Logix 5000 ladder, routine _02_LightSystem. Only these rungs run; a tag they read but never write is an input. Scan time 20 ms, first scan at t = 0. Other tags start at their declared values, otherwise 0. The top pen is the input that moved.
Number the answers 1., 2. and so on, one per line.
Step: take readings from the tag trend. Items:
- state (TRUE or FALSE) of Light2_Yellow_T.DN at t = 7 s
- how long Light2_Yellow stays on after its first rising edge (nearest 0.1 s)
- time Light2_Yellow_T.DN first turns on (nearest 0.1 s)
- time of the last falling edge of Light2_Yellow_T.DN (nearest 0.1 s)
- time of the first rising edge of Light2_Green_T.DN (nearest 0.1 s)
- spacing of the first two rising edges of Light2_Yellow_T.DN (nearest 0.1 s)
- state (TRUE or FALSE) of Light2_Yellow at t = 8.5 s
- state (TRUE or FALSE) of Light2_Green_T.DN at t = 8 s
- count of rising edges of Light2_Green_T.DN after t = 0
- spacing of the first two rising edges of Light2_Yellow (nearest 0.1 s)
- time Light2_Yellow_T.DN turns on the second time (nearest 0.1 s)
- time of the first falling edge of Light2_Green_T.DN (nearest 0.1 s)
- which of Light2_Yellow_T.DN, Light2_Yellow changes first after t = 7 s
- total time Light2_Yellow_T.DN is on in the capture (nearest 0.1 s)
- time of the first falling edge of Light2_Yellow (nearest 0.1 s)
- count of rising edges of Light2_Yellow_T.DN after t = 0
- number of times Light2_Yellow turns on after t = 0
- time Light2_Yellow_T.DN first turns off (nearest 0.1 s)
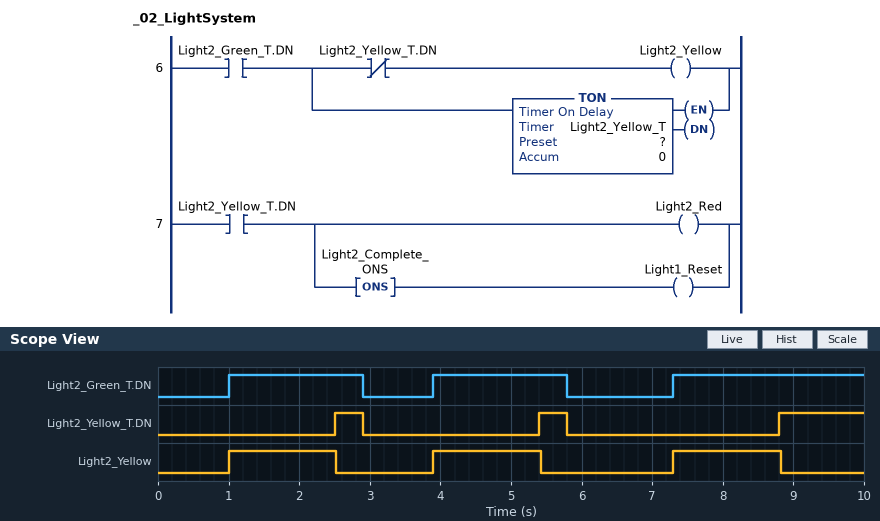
1. FALSE
2. 1.5 s
3. 2.5 s
4. 5.8 s
5. 1.0 s
6. 2.9 s
7. TRUE
8. TRUE
9. 3
10. 2.9 s
11. 5.4 s
12. 2.9 s
13. Light2_Yellow
14. 2.0 s
15. 2.5 s
16. 3
17. 3
18. 2.9 s
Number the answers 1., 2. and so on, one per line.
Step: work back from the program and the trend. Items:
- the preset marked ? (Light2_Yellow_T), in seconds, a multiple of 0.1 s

1. 1.5 s
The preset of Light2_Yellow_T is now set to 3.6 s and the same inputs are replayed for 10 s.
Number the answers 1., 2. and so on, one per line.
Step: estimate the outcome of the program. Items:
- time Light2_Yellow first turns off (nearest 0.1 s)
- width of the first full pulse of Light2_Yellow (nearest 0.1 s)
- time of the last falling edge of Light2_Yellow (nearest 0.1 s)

1. 2.9 s
2. 1.9 s
3. 5.8 s
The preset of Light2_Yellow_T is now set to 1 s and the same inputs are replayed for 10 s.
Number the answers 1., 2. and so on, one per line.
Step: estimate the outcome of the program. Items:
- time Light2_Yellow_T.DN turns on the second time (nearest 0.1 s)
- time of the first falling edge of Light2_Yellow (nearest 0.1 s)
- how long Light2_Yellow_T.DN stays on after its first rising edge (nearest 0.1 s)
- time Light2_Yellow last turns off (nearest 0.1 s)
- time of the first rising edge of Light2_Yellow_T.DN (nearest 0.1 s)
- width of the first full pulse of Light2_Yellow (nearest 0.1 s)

1. 4.9 s
2. 2.0 s
3. 0.9 s
4. 8.3 s
5. 2.0 s
6. 1.0 s
